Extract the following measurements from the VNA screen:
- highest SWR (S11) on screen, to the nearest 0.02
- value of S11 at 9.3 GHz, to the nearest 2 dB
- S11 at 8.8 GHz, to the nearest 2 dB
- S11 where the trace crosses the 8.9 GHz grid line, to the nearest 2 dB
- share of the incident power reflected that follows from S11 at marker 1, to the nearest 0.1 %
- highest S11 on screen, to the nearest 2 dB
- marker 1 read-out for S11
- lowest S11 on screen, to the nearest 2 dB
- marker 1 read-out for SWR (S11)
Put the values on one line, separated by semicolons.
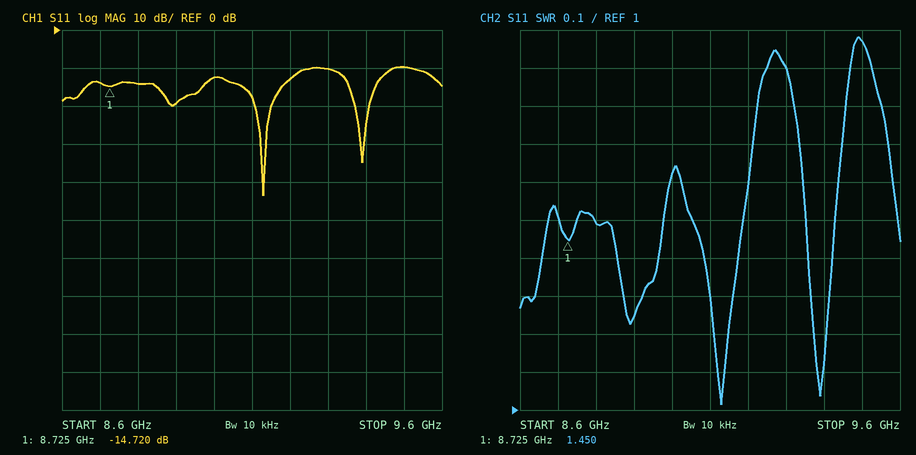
1.98; -10 dB; -14 dB; -20 dB; 3.4 %; -10 dB; -14.720 dB; -44 dB; 1.450
